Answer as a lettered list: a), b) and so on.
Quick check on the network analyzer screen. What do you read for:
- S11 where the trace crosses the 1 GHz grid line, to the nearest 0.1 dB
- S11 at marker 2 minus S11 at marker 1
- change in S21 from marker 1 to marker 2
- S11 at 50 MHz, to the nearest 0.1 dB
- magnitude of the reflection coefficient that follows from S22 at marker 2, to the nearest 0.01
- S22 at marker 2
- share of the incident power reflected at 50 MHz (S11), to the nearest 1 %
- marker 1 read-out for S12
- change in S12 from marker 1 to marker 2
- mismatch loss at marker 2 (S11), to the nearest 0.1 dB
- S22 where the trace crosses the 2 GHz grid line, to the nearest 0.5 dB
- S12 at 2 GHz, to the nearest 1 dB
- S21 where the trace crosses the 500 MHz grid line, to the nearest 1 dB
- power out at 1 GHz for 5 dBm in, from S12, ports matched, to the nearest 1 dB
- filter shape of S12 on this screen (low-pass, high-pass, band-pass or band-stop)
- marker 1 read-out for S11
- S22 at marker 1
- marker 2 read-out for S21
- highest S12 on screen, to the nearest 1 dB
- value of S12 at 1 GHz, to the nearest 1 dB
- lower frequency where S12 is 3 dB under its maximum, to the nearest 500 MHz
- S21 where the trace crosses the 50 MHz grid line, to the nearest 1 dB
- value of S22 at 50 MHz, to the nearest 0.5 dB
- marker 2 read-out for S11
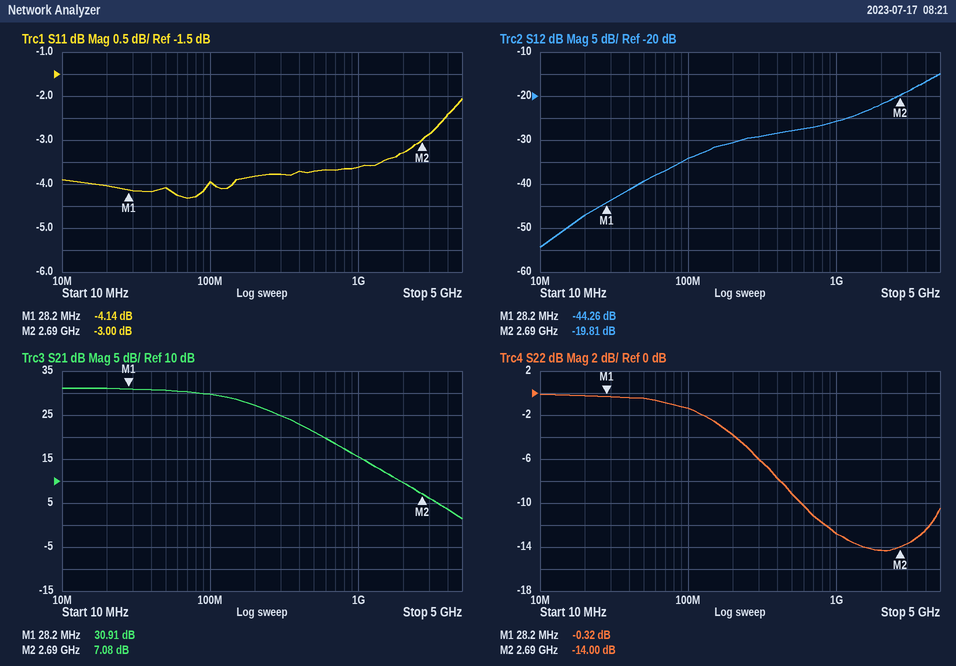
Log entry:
a) -3.6 dB
b) 1.14 dB
c) -23.83 dB
d) -4.1 dB
e) 0.20
f) -14.00 dB
g) 39 %
h) -44.26 dB
i) 24.45 dB
j) 3.0 dB
k) -14.5 dB
l) -22 dB
m) 21 dB
n) -21 dBm
o) high-pass
p) -4.14 dB
q) -0.32 dB
r) 7.08 dB
s) -15 dB
t) -26 dB
u) 3.5 GHz
v) 31 dB
w) -0.5 dB
x) -3.00 dB
